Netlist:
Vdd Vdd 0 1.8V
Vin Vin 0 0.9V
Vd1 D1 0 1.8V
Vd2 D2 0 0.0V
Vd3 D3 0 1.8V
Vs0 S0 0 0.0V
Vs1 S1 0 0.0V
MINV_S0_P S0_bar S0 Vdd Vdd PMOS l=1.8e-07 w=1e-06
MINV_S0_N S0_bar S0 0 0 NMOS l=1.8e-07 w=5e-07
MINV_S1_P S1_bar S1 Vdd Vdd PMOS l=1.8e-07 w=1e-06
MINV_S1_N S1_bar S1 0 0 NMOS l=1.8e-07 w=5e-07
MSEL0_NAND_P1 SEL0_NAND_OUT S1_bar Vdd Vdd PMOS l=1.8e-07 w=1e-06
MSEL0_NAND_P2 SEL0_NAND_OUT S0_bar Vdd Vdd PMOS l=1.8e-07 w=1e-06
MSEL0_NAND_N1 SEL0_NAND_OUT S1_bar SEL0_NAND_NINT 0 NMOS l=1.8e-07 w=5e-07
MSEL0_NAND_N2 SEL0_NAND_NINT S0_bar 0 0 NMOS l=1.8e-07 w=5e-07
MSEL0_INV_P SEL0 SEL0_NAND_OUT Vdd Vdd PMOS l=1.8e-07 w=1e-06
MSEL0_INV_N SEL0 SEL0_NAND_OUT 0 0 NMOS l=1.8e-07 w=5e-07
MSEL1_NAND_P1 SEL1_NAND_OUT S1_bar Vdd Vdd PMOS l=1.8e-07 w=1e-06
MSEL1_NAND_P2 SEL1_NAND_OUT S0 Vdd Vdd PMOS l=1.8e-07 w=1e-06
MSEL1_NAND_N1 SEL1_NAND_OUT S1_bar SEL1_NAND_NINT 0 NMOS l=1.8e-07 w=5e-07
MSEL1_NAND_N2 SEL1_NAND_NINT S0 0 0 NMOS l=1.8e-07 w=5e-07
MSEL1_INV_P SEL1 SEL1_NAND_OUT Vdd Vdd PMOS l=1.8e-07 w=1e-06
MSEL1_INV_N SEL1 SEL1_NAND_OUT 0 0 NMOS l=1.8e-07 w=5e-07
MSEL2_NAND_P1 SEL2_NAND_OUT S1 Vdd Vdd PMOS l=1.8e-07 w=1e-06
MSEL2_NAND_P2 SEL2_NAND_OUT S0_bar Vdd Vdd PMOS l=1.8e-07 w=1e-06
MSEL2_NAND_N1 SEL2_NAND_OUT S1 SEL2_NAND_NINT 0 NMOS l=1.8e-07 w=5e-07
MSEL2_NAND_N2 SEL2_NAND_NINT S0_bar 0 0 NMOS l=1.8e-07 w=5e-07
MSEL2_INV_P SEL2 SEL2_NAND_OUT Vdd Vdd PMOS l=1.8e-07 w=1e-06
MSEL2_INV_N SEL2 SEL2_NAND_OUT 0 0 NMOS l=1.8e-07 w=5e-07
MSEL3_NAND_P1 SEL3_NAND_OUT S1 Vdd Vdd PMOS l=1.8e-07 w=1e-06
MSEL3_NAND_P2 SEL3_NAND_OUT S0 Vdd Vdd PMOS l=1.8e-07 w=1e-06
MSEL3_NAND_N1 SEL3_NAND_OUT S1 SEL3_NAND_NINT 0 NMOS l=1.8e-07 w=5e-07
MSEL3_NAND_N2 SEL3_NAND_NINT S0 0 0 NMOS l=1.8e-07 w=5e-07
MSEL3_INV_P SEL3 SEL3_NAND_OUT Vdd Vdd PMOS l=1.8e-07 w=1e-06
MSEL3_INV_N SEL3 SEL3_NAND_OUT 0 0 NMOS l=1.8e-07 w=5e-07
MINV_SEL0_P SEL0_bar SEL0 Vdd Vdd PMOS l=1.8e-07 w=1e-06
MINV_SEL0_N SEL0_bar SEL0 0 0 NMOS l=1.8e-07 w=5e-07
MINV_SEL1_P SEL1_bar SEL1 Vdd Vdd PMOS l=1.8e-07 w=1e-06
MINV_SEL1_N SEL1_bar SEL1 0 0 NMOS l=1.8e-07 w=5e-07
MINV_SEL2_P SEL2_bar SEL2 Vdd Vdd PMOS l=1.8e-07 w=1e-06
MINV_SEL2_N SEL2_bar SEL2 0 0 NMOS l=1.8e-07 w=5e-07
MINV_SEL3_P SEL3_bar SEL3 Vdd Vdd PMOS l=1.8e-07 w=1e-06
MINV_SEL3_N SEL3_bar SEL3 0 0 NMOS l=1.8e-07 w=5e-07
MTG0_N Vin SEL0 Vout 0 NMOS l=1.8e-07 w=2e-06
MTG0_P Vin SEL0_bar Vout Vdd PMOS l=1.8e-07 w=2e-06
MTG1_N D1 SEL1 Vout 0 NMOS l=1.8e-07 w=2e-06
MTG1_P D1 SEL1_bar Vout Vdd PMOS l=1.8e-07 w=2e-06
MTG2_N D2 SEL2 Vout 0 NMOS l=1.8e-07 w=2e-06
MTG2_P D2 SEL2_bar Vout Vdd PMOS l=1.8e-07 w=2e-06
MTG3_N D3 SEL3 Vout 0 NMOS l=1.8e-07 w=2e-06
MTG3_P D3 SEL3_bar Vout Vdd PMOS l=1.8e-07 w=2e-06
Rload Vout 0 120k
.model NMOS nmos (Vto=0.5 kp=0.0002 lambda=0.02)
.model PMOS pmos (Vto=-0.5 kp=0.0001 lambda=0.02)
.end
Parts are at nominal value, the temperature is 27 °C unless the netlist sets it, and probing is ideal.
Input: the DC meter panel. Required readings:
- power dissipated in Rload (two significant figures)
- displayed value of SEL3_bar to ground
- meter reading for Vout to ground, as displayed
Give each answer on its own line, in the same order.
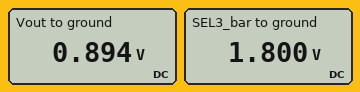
6.7 µW
1.800 V
0.894 V
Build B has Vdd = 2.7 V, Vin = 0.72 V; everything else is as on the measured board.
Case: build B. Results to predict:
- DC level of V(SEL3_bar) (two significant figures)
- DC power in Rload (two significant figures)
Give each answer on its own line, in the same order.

2.7 V
4.3 µW
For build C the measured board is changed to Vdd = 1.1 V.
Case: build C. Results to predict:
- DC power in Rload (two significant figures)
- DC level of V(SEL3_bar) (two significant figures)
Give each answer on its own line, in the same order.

7.9 µW
1.1 V
